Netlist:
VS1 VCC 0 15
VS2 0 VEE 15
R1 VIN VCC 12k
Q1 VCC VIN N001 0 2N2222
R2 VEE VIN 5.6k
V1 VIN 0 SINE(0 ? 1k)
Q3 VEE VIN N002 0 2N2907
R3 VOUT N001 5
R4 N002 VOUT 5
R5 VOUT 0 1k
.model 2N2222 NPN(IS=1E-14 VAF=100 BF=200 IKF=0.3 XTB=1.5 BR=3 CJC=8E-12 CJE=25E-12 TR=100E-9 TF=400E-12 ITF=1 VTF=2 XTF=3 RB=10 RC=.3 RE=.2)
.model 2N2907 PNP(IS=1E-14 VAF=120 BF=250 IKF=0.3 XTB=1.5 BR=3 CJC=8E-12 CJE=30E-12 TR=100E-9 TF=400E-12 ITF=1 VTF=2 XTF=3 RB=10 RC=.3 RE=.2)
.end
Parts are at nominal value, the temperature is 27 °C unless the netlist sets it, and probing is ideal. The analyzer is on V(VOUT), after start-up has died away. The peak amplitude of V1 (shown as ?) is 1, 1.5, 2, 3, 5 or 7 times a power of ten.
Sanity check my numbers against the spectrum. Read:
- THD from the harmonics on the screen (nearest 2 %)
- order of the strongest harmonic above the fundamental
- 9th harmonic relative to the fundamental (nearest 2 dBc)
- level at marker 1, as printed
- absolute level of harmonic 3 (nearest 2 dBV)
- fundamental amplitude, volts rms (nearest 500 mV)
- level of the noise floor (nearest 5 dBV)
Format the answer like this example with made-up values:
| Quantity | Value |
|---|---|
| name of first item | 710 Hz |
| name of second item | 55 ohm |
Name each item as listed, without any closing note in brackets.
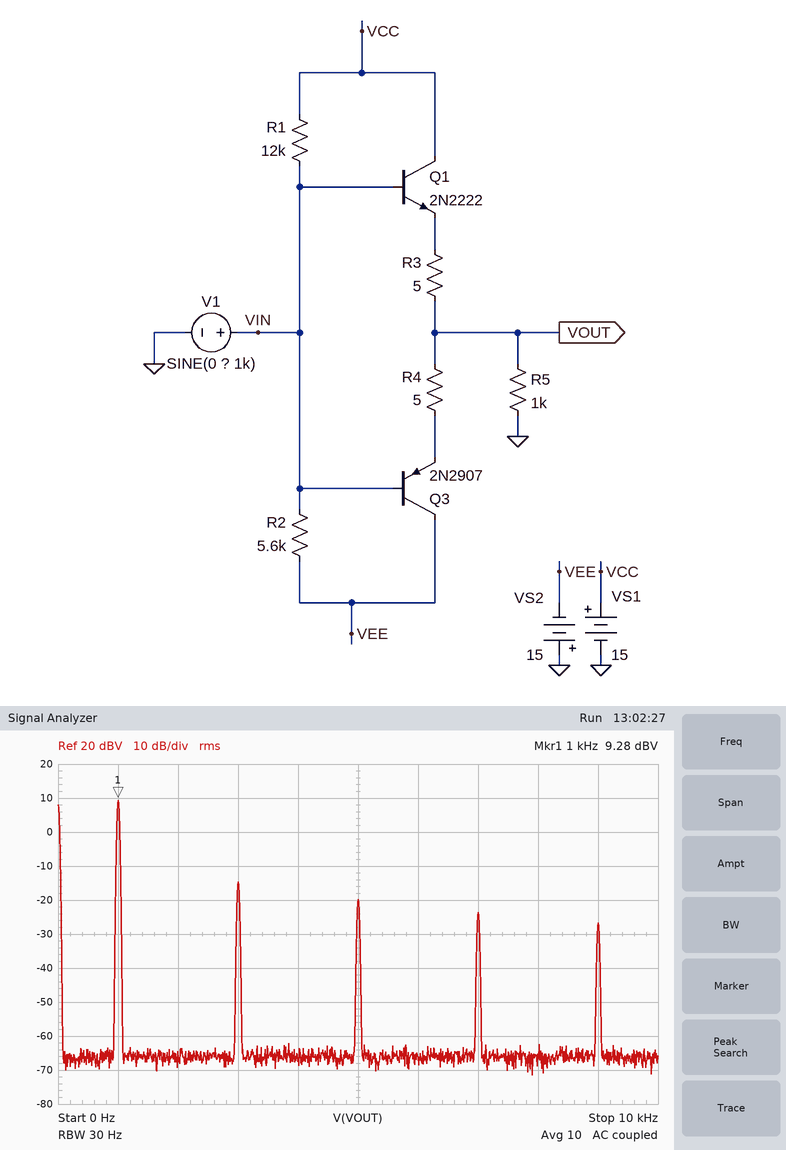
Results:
| Quantity | Value |
|---|---|
| THD from the harmonics on the screen | 8 % |
| order of the strongest harmonic above the fundamental | 3 |
| 9th harmonic relative to the fundamental | -36 dBc |
| level at marker 1, as printed | 9.28 dBV |
| absolute level of harmonic 3 | -14 dBV |
| fundamental amplitude, volts rms | 3.0 V |
| level of the noise floor | -65 dBV |
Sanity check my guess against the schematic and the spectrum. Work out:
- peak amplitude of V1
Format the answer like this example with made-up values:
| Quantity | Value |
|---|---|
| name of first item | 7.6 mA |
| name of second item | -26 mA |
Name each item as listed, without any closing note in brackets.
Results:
| Quantity | Value |
|---|---|
| peak amplitude of V1 | 5 V |
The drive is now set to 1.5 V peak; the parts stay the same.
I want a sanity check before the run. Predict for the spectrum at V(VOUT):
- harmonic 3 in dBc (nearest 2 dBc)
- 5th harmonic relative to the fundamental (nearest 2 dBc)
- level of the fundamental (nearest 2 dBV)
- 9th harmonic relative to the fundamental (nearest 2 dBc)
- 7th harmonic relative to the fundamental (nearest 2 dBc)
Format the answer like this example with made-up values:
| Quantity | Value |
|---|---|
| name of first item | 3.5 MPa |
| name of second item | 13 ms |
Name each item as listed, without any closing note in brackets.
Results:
| Quantity | Value |
|---|---|
| harmonic 3 in dBc | -12 dBc |
| 5th harmonic relative to the fundamental | -22 dBc |
| level of the fundamental | -6 dBV |
| 9th harmonic relative to the fundamental | -40 dBc |
| 7th harmonic relative to the fundamental | -36 dBc |
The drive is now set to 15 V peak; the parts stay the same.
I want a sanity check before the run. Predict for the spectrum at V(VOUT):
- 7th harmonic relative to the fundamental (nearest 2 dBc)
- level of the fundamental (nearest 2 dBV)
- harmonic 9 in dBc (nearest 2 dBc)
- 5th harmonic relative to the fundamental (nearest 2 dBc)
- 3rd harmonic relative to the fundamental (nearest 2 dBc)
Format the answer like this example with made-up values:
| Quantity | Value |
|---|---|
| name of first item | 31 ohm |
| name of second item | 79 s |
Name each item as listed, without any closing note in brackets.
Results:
| Quantity | Value |
|---|---|
| 7th harmonic relative to the fundamental | -42 dBc |
| level of the fundamental | 20 dBV |
| harmonic 9 in dBc | -44 dBc |
| 5th harmonic relative to the fundamental | -38 dBc |
| 3rd harmonic relative to the fundamental | -34 dBc |
